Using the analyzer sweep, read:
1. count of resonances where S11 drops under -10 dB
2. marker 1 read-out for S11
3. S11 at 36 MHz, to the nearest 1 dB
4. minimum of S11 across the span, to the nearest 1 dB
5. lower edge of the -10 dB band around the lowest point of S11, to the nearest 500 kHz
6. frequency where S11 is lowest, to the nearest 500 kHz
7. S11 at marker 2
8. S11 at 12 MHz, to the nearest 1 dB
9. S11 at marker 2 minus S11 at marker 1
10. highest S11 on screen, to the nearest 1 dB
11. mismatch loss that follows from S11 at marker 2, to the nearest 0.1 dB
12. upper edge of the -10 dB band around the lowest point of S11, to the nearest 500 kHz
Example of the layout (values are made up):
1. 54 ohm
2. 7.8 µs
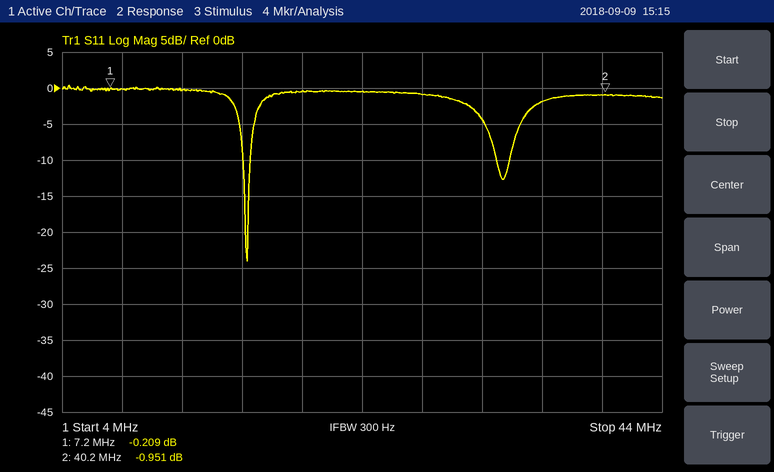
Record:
1. 2
2. -0.209 dB
3. -2 dB
4. -24 dB
5. 16.0 MHz
6. 16.5 MHz
7. -0.951 dB
8. 0 dB
9. -0.742 dB
10. 0 dB
11. 7.1 dB
12. 16.5 MHz
